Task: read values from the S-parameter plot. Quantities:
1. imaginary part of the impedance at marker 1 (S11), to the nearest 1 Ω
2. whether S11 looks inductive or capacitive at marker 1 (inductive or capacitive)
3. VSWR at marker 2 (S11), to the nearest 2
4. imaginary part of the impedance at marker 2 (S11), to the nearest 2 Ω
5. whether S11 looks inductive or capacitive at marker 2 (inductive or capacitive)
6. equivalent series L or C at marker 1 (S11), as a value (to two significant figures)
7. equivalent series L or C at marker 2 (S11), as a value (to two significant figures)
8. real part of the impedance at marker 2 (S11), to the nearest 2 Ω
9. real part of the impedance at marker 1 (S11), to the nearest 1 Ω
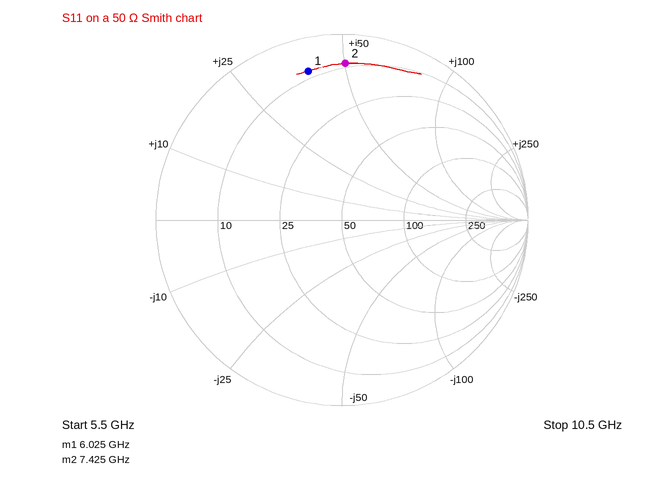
+39 Ω
inductive
12
+50 Ω
inductive
1.0 nH
1.1 nH
8 Ω
8 Ω
